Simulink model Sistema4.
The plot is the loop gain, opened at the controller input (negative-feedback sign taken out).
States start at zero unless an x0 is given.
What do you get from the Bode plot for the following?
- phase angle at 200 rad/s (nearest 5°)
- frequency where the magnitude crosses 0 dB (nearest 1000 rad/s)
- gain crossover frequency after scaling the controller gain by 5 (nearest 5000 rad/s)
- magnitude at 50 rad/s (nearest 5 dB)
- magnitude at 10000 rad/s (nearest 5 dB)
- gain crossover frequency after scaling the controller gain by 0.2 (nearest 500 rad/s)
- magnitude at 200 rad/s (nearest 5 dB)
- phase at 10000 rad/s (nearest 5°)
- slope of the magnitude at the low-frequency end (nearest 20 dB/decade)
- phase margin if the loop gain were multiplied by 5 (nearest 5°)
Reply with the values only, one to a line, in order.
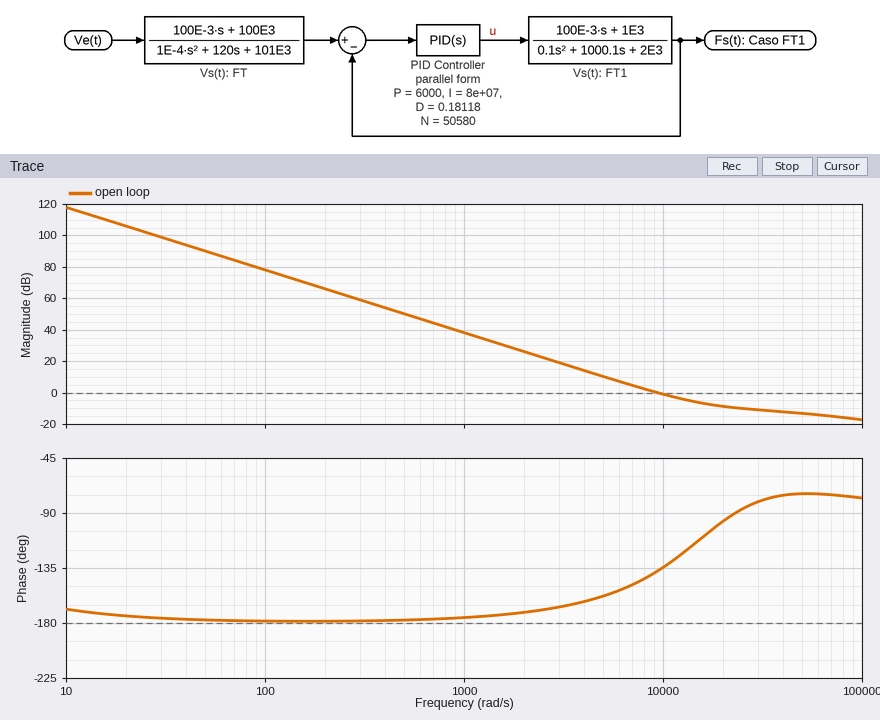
-180°
9000 rad/s
60000 rad/s
90 dB
0 dB
4000 rad/s
65 dB
-135°
-40 dB/decade
105°
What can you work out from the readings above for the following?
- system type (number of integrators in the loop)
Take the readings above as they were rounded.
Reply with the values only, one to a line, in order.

2
